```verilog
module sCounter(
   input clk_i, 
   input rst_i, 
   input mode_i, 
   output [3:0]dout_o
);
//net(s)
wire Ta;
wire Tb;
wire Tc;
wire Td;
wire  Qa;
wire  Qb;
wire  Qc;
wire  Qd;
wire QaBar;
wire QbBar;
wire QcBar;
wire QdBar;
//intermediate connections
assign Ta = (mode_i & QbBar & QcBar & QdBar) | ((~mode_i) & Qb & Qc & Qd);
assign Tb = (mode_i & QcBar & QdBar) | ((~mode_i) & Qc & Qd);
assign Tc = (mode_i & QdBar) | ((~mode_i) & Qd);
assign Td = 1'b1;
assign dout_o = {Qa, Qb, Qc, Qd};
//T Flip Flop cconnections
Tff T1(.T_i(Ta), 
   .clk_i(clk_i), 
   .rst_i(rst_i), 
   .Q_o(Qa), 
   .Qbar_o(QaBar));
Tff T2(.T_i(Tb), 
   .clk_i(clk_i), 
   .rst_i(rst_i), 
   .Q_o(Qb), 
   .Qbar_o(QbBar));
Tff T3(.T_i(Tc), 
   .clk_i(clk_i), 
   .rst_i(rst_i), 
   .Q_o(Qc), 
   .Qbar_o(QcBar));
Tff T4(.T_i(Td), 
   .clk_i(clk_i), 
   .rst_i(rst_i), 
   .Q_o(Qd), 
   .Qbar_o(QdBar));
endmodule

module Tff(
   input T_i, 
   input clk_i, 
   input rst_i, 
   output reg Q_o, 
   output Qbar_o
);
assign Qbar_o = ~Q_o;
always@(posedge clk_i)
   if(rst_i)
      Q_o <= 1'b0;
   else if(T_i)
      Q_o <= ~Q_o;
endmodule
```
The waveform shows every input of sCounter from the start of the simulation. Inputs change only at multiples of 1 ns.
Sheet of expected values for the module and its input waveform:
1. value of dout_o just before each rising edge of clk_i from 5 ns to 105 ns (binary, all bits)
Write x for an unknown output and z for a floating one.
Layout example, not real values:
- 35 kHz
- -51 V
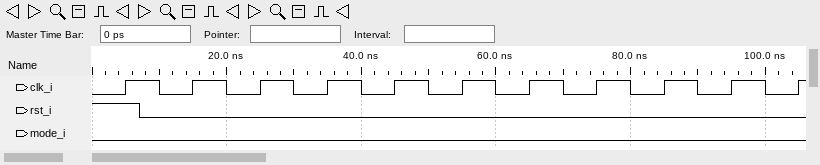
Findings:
- x, 0000, 0001, 0010, 0011, 0100, 0101, 0110, 0111, 1000, 1001
